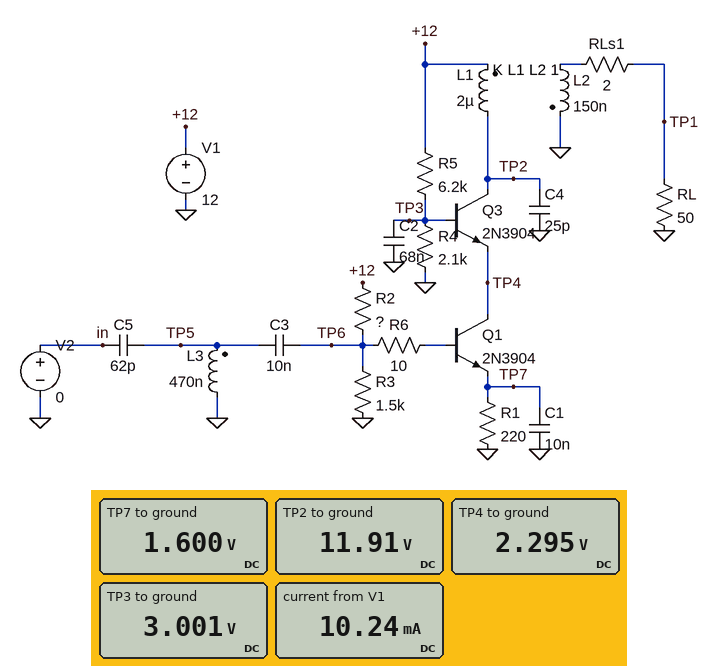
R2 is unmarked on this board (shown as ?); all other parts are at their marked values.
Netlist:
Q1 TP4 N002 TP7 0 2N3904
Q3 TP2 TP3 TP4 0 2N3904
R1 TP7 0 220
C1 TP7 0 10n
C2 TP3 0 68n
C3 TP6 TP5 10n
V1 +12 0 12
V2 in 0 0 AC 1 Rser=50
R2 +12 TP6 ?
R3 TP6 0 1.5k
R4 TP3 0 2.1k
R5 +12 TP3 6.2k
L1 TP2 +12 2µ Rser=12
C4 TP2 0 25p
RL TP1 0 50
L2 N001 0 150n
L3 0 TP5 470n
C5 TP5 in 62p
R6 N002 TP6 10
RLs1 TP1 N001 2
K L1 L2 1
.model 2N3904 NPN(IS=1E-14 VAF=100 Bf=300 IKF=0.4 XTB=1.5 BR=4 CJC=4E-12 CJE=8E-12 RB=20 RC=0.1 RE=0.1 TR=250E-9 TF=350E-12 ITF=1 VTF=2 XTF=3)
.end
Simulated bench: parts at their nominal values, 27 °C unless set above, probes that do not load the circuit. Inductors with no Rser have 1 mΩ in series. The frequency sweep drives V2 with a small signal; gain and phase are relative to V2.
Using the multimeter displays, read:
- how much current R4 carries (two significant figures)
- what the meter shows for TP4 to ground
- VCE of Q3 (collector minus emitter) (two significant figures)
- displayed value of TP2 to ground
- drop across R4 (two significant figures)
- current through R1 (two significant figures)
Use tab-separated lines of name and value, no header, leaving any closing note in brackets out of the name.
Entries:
how much current R4 carries	1.4 mA
what the meter shows for TP4 to ground	2.295 V
VCE of Q3 (collector minus emitter)	9.6 V
displayed value of TP2 to ground	11.91 V
drop across R4	3.0 V
current through R1	7.3 mA
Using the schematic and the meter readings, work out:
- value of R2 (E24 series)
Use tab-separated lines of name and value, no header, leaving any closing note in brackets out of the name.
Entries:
value of R2	6.2 kΩ
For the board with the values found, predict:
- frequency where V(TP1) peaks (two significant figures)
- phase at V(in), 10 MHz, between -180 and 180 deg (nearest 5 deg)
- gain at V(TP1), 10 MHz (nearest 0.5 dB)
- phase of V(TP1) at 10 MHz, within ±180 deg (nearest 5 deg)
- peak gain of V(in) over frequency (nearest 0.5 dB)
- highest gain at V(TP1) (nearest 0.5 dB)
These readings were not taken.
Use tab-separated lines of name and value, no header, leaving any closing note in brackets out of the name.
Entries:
frequency where V(TP1) peaks	19 MHz
phase at V(in), 10 MHz, between -180 and 180 deg	-15 deg
gain at V(TP1), 10 MHz	4.5 dB
phase of V(TP1) at 10 MHz, within ±180 deg	70 deg
peak gain of V(in) over frequency	0 dB
highest gain at V(TP1)	32.0 dB
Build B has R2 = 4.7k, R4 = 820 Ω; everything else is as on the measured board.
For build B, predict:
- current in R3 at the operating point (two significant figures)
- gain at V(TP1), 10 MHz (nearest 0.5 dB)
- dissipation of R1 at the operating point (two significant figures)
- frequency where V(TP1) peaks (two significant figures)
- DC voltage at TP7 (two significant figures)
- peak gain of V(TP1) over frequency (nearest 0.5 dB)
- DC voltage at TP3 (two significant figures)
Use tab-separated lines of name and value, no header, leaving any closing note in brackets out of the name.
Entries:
current in R3 at the operating point	970 µA
gain at V(TP1), 10 MHz	-32.0 dB
dissipation of R1 at the operating point	2.3 mW
frequency where V(TP1) peaks	22 MHz
DC voltage at TP7	710 mV
peak gain of V(TP1) over frequency	-13.5 dB
DC voltage at TP3	1.4 V
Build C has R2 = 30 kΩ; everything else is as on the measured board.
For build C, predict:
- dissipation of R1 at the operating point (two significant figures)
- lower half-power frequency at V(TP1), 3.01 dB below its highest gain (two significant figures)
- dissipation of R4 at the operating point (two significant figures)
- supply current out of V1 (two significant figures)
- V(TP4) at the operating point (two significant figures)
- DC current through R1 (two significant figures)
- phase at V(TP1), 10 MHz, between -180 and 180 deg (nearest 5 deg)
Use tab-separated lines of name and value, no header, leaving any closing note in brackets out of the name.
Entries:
dissipation of R1 at the operating point	210 nW
lower half-power frequency at V(TP1), 3.01 dB below its highest gain	20 MHz
dissipation of R4 at the operating point	4.4 mW
supply current out of V1	1.9 mA
V(TP4) at the operating point	2.5 V
DC current through R1	31 µA
phase at V(TP1), 10 MHz, between -180 and 180 deg	15 deg
